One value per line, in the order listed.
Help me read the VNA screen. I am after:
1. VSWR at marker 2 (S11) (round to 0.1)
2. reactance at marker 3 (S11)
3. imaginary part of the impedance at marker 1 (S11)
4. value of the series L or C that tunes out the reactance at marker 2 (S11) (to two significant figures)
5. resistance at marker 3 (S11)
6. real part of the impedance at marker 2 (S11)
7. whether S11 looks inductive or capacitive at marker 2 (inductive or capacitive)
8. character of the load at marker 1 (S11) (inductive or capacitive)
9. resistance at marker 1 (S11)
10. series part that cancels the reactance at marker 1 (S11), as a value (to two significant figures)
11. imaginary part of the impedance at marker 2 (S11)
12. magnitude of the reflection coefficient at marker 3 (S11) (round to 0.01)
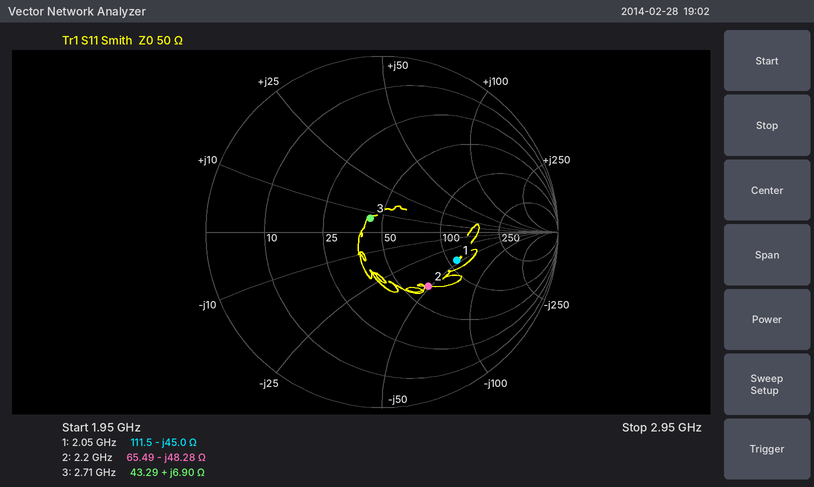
2.4
+6.90 Ω
-45.0 Ω
3.5 nH
43.29 Ω
65.49 Ω
capacitive
capacitive
111.5 Ω
3.5 nH
-48.28 Ω
0.10
